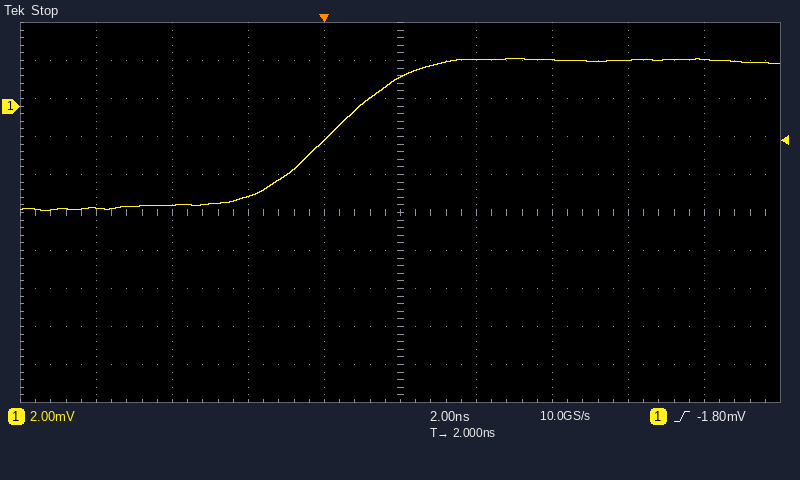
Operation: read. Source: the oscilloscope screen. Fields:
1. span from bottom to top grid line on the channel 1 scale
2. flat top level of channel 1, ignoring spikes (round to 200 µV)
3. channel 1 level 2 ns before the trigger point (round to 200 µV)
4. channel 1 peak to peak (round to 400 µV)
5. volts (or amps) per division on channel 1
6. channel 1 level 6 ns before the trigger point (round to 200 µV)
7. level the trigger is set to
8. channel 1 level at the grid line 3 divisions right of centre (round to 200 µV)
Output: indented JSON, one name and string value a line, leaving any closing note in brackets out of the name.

{
  "span from bottom to top grid line on the channel 1 scale": "20 mV",
  "flat top level of channel 1, ignoring spikes": "2.4 mV",
  "channel 1 level 2 ns before the trigger point": "-4.8 mV",
  "channel 1 peak to peak": "8.0 mV",
  "volts (or amps) per division on channel 1": "2 mV",
  "channel 1 level 6 ns before the trigger point": "-5.4 mV",
  "level the trigger is set to": "-1.80 mV",
  "channel 1 level at the grid line 3 divisions right of centre": "2.4 mV"
}
